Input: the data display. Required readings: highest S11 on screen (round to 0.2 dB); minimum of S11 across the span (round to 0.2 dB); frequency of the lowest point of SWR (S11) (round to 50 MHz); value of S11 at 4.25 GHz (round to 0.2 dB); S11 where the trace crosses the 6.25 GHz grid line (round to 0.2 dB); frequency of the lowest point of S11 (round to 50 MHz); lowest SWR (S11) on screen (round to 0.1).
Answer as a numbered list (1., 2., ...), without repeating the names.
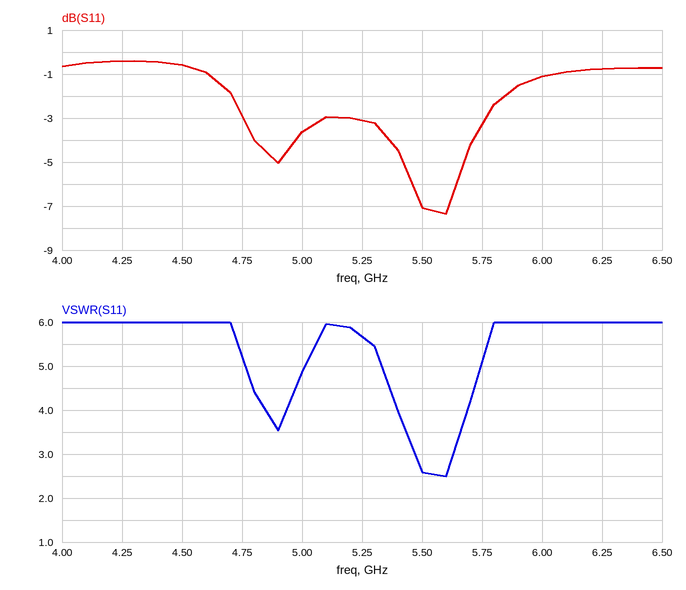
1. -0.4 dB
2. -7.4 dB
3. 5.60 GHz
4. -0.4 dB
5. -0.8 dB
6. 5.60 GHz
7. 2.5
